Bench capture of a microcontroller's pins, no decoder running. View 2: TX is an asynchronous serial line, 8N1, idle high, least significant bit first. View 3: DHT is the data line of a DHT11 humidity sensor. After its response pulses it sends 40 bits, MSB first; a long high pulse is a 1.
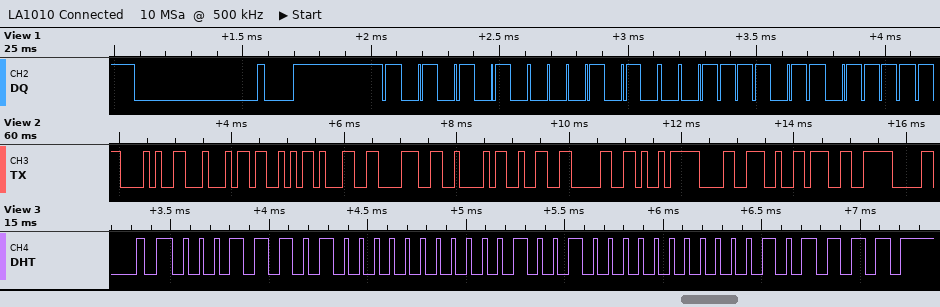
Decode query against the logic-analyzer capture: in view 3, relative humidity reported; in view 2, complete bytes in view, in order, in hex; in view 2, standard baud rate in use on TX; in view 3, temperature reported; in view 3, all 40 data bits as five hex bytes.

29 %
0x28 0x44 0x53 0x31 0x38 0x42 0x32 0x30 0xE9 0x98 0xB2 0xE6
9600 baud
18.0 °C
1D 00 12 00 2F
